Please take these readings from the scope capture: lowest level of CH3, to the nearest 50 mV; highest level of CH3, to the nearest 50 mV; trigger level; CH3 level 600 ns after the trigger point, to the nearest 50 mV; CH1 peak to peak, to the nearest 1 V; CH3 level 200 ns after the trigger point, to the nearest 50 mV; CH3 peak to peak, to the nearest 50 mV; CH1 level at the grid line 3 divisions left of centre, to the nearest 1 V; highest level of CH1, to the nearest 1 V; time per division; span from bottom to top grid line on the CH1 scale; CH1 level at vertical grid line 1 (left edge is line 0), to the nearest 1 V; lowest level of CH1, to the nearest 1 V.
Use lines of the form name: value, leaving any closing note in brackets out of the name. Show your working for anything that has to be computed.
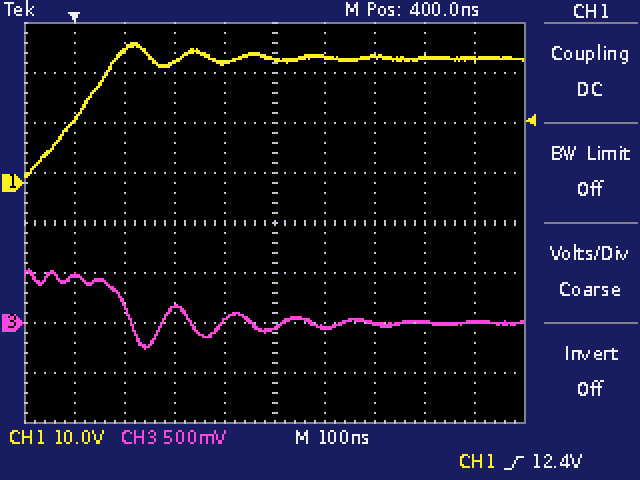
lowest level of CH3, to the nearest 50 mV: -250 mV
highest level of CH3, to the nearest 50 mV: 550 mV
trigger level: 12.4 V
CH3 level 600 ns after the trigger point, to the nearest 50 mV: 0 mV
CH1 peak to peak, to the nearest 1 V: 28 V − (1 V) = 27 V
CH3 level 200 ns after the trigger point, to the nearest 50 mV: 150 mV
CH3 peak to peak, to the nearest 50 mV: 550 mV − (-250 mV) = 800 mV
CH1 level at the grid line 3 divisions left of centre, to the nearest 1 V: 27 V
highest level of CH1, to the nearest 1 V: 28 V
time per division: 100 ns
span from bottom to top grid line on the CH1 scale: 80 V
CH1 level at vertical grid line 1 (left edge is line 0), to the nearest 1 V: 13 V
lowest level of CH1, to the nearest 1 V: 1 V
